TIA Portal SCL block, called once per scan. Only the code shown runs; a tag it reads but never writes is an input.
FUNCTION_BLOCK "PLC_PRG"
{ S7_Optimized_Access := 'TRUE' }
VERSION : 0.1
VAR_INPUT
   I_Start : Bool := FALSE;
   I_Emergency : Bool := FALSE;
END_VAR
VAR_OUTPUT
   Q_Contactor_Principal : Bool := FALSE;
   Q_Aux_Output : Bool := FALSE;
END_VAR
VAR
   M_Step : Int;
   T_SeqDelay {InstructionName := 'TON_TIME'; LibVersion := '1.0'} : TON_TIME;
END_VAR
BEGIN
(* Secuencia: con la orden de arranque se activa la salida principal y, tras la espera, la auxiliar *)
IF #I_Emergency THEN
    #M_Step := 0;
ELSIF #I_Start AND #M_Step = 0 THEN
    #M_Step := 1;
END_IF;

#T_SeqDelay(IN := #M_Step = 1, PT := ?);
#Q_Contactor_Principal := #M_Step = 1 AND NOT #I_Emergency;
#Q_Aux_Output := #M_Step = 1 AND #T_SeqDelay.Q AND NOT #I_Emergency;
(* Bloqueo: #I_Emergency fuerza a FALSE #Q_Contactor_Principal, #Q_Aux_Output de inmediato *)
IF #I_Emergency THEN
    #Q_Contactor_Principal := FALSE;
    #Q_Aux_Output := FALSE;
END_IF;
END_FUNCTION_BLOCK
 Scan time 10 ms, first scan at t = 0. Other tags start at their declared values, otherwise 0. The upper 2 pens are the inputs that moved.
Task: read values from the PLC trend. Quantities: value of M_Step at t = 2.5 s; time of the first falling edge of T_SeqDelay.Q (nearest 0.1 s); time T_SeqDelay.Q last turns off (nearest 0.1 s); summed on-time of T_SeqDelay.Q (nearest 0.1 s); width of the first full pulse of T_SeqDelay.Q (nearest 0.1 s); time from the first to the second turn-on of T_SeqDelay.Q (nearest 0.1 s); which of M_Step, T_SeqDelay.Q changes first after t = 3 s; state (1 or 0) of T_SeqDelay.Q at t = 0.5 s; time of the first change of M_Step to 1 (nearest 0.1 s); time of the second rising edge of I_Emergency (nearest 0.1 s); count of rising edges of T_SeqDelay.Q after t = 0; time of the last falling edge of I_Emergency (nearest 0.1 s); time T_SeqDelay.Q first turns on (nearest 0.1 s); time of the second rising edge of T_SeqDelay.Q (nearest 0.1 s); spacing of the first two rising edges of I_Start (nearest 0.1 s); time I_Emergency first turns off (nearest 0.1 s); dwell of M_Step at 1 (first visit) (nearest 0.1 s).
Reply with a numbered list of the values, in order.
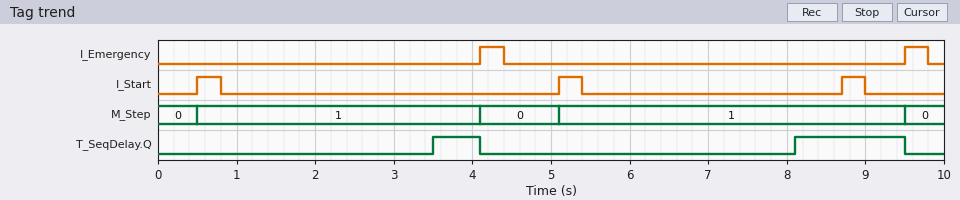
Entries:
1. 1
2. 4.1 s
3. 9.5 s
4. 2.0 s
5. 0.6 s
6. 4.6 s
7. T_SeqDelay.Q
8. 0
9. 0.5 s
10. 9.5 s
11. 2
12. 9.8 s
13. 3.5 s
14. 8.1 s
15. 4.6 s
16. 4.4 s
17. 3.6 s
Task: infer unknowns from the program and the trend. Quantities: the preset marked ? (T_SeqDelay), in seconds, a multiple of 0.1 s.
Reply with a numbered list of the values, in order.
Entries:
1. 3.0 s
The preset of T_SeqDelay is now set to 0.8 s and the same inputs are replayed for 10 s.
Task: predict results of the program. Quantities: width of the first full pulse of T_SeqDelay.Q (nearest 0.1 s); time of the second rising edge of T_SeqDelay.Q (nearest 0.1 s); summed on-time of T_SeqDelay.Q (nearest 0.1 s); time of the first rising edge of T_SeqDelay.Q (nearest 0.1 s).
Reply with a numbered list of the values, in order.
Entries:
1. 2.8 s
2. 5.9 s
3. 6.4 s
4. 1.3 s
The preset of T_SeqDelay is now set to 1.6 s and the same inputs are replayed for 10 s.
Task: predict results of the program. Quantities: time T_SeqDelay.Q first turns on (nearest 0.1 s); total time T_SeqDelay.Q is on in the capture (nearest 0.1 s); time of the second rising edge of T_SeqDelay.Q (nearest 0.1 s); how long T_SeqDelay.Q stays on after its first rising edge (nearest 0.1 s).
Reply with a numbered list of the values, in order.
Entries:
1. 2.1 s
2. 4.8 s
3. 6.7 s
4. 2.0 s
